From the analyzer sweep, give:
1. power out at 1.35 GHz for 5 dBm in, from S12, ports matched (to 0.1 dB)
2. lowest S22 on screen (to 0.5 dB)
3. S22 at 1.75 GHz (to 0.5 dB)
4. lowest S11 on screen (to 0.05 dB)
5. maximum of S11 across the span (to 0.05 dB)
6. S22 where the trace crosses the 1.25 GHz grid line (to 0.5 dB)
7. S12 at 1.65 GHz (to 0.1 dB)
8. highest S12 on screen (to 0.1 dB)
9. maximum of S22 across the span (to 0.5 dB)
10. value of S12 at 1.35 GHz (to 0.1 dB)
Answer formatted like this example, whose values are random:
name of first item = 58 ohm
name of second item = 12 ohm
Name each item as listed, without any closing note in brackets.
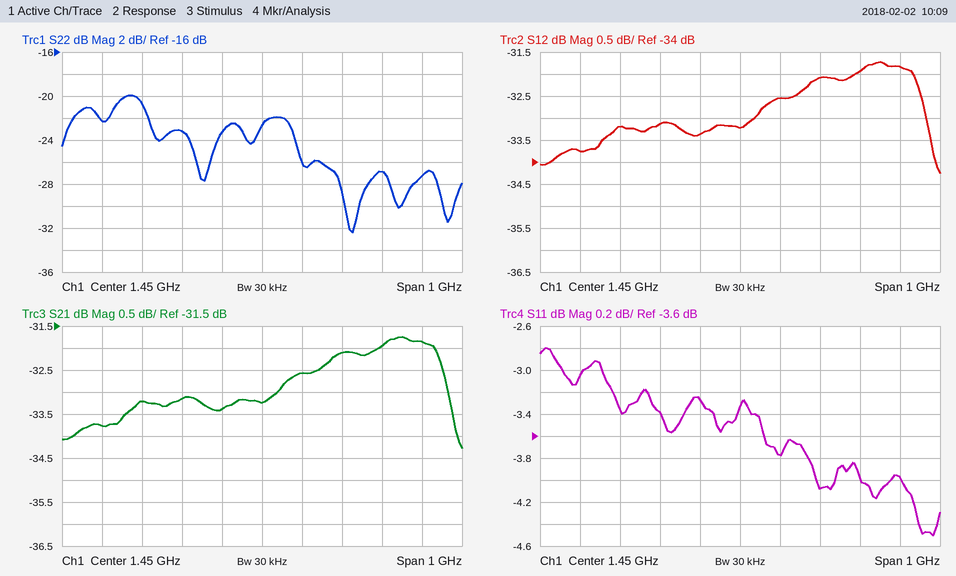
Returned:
power out at 1.35 GHz for 5 dBm in, from S12, ports matched = -28.4 dBm
lowest S22 on screen = -32.5 dB
S22 at 1.75 GHz = -27.0 dB
lowest S11 on screen = -4.50 dB
maximum of S11 across the span = -2.80 dB
S22 where the trace crosses the 1.25 GHz grid line = -23.0 dB
S12 at 1.65 GHz = -32.1 dB
highest S12 on screen = -31.7 dB
maximum of S22 across the span = -20.0 dB
value of S12 at 1.35 GHz = -33.4 dB
